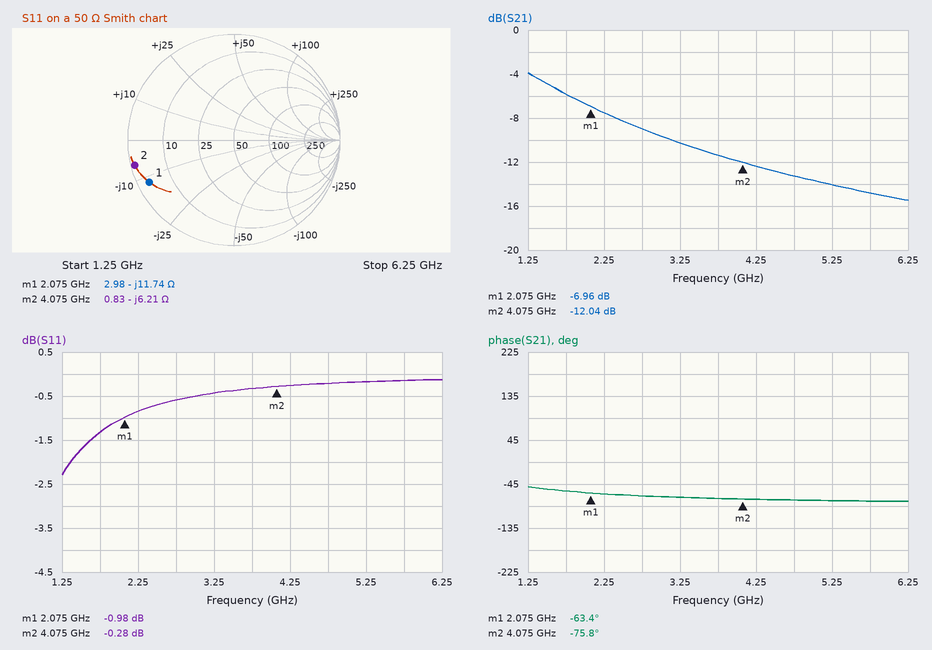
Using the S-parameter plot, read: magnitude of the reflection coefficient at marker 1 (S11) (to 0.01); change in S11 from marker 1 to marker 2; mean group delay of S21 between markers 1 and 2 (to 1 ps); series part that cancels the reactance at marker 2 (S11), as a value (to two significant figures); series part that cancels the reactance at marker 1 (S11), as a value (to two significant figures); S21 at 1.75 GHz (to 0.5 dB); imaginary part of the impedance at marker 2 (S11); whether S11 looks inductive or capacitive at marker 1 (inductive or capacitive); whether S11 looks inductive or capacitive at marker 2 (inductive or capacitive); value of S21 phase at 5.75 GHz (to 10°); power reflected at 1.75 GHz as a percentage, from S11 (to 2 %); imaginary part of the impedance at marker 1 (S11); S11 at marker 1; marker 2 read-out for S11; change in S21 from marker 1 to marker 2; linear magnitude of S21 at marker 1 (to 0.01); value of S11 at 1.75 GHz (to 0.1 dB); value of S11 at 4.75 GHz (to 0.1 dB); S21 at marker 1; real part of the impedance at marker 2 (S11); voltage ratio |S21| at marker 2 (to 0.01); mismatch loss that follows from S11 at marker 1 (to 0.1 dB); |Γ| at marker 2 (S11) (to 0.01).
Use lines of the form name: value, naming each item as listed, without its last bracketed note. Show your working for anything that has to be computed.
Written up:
magnitude of the reflection coefficient at marker 1 (S11): 0.89
change in S11 from marker 1 to marker 2: -0.28 − (-0.98) = 0.70 dB
mean group delay of S21 between markers 1 and 2: −(-75.8° − (-63.4°))/(360° × 2 GHz) ≈ 17 ps
series part that cancels the reactance at marker 2 (S11), as a value: L = 6.21 Ω/(2π × 4.075 GHz) ≈ 243 pH, so 240 pH to two significant figures
series part that cancels the reactance at marker 1 (S11), as a value: L = 11.74 Ω/(2π × 2.075 GHz) ≈ 900 pH
S21 at 1.75 GHz: -6.0 dB
imaginary part of the impedance at marker 2: -6.21 Ω
whether S11 looks inductive or capacitive at marker 1: capacitive
whether S11 looks inductive or capacitive at marker 2: capacitive
value of S21 phase at 5.75 GHz: -80°
power reflected at 1.75 GHz as a percentage, from S11: 10^(-1.3/10) ≈ 74 %
imaginary part of the impedance at marker 1: -11.74 Ω
S11 at marker 1: -0.98 dB
marker 2 read-out for S11: -0.28 dB
change in S21 from marker 1 to marker 2: -12.04 − (-6.96) = -5.08 dB
linear magnitude of S21 at marker 1: 10^(-6.96/20) ≈ 0.45
value of S11 at 1.75 GHz: -1.3 dB
value of S11 at 4.75 GHz: -0.2 dB
S21 at marker 1: -6.96 dB
real part of the impedance at marker 2: 0.83 Ω
voltage ratio |S21| at marker 2: 10^(-12.04/20) ≈ 0.25
mismatch loss that follows from S11 at marker 1: −10 log10(1 − 10^(-0.98/10)) ≈ 6.9 dB
|Γ| at marker 2 (S11): 0.97
